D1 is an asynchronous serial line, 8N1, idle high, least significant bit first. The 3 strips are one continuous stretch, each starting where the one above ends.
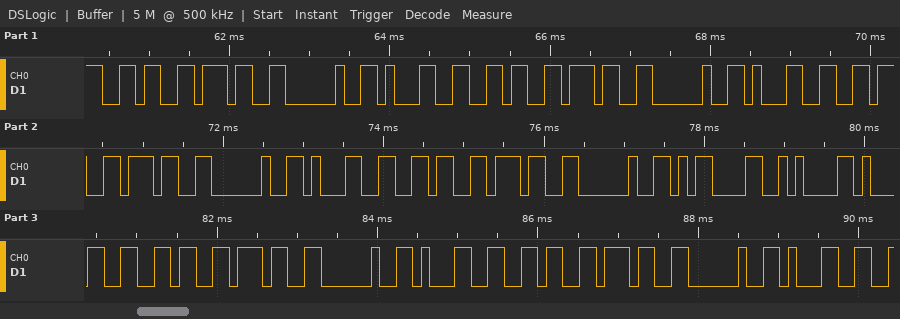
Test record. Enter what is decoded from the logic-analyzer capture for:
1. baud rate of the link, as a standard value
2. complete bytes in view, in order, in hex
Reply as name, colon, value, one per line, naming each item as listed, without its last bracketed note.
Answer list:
baud rate of the link, as a standard value: 9600 baud
complete bytes in view, in order, in hex: 0x36 0x37 0x20 0x31 0x36 0x37 0x20 0x31 0x36 0x37 0x20 0x31 0x36 0x37 0x20 0x0D 0x0A 0x31 0x36 0x37 0x20 0x31 0x36 0x37 0x20 0x31
